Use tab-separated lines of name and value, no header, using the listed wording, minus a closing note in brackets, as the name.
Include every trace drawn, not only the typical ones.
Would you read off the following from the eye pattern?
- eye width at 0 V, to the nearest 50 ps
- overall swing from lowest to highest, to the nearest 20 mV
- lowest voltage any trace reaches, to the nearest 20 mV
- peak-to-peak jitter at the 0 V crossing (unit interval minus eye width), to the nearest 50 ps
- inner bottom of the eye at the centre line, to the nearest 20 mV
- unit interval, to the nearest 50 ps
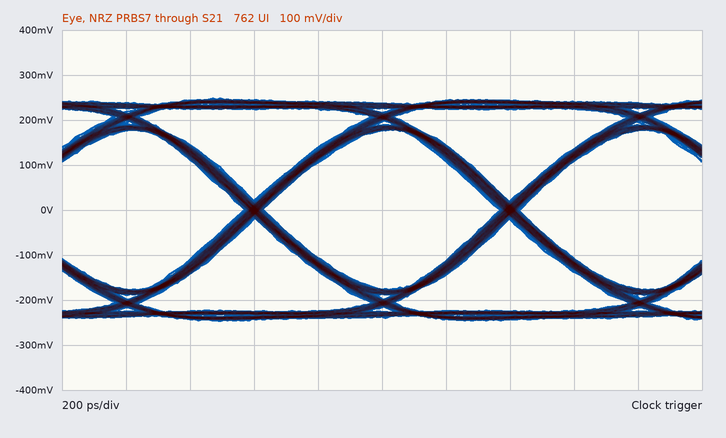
eye width at 0 V, to the nearest 50 ps	750 ps
overall swing from lowest to highest, to the nearest 20 mV	500 mV
lowest voltage any trace reaches, to the nearest 20 mV	-240 mV
peak-to-peak jitter at the 0 V crossing (unit interval minus eye width), to the nearest 50 ps	50 ps
inner bottom of the eye at the centre line, to the nearest 20 mV	-180 mV
unit interval, to the nearest 50 ps	800 ps
